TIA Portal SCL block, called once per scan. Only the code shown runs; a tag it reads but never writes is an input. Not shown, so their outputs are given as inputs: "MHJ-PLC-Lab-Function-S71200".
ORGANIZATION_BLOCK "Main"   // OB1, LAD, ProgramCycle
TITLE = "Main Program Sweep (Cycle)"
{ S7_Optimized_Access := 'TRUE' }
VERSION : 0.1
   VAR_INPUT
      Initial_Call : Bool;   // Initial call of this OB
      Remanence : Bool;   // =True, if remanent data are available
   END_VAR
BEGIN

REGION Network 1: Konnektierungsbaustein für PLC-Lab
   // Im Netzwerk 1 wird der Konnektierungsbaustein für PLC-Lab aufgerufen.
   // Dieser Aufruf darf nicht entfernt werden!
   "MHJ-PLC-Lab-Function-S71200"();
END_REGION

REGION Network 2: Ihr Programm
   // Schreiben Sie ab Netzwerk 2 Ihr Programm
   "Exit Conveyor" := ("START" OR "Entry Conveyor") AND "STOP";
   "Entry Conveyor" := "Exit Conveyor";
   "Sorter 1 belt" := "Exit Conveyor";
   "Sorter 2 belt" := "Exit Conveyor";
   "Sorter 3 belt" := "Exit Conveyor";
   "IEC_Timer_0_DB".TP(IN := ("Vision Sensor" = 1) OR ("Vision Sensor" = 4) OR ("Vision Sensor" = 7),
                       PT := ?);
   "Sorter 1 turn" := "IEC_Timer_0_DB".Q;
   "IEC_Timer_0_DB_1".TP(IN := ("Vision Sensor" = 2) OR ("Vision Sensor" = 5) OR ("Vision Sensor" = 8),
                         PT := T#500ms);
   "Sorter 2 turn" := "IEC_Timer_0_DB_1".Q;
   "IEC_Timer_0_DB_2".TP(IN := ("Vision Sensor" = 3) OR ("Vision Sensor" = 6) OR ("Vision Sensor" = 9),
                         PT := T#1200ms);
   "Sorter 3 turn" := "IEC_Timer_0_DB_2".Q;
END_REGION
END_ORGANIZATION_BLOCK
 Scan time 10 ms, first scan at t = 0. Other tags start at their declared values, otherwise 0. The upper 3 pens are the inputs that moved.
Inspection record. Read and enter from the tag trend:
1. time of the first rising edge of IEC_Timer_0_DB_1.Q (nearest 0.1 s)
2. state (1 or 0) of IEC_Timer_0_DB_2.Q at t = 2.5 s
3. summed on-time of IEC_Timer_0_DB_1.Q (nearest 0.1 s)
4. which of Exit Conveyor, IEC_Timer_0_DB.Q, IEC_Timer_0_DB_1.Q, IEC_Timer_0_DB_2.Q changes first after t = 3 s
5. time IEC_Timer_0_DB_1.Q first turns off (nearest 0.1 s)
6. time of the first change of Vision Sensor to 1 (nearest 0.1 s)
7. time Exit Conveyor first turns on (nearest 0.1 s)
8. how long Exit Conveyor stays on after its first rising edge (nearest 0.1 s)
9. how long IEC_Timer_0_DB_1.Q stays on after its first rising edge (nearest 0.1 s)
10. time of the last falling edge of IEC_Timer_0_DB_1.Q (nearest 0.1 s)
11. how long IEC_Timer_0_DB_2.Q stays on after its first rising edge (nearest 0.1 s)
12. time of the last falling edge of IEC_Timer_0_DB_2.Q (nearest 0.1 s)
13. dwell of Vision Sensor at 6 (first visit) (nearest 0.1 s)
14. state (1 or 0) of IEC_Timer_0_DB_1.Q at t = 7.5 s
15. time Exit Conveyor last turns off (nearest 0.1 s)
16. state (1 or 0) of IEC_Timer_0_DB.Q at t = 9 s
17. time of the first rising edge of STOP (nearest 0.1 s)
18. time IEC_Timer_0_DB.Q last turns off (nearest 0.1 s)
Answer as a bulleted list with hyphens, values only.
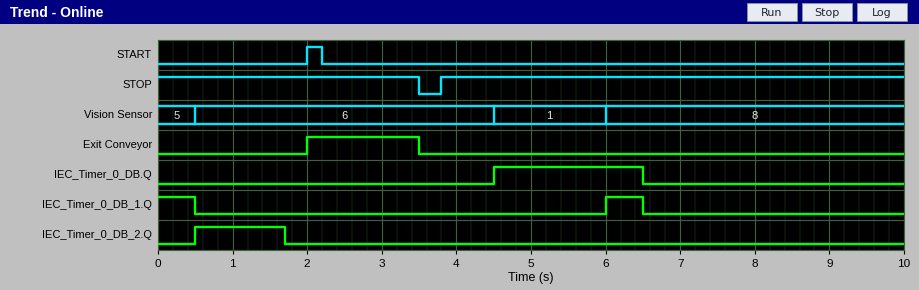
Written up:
- 6.0 s
- 0
- 1.0 s
- Exit Conveyor
- 0.5 s
- 4.5 s
- 2.0 s
- 1.5 s
- 0.5 s
- 6.5 s
- 1.2 s
- 1.7 s
- 4.0 s
- 0
- 3.5 s
- 0
- 3.8 s
- 6.5 s
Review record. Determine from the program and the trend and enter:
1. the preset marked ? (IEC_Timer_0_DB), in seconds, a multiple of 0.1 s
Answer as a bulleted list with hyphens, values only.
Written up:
- 2.0 s
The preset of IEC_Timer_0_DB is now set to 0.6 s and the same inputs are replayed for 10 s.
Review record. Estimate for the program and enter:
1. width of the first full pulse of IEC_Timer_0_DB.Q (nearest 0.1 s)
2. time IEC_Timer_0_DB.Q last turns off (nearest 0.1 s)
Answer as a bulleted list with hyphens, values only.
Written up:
- 0.6 s
- 5.1 s
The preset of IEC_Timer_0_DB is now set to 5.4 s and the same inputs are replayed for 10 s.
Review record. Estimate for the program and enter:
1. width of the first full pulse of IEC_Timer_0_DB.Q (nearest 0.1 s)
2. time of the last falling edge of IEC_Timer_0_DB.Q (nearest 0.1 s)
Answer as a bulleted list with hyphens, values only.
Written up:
- 5.4 s
- 9.9 s
